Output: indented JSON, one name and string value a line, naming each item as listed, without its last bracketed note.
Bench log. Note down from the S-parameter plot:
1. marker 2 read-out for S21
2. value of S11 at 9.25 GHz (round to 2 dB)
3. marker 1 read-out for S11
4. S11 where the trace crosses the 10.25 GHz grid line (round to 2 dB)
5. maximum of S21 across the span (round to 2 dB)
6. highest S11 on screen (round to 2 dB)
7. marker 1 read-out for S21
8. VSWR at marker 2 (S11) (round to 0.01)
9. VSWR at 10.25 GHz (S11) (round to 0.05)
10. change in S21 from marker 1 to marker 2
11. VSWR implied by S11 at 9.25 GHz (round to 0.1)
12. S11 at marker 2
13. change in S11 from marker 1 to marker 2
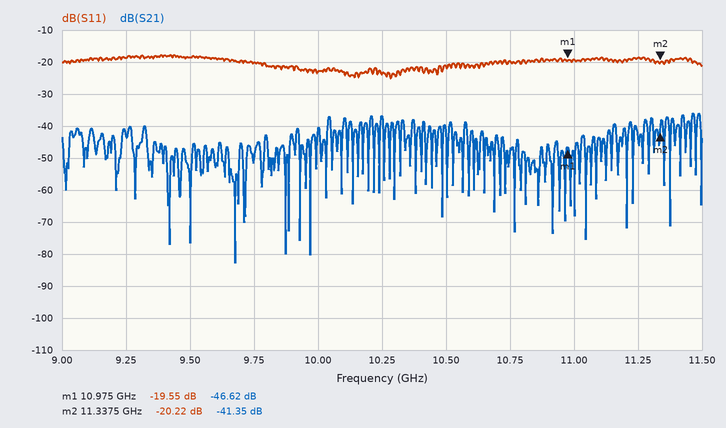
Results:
{
  "marker 2 read-out for S21": "-41.35 dB",
  "value of S11 at 9.25 GHz": "-18 dB",
  "marker 1 read-out for S11": "-19.55 dB",
  "S11 where the trace crosses the 10.25 GHz grid line": "-24 dB",
  "maximum of S21 across the span": "-36 dB",
  "highest S11 on screen": "-18 dB",
  "marker 1 read-out for S21": "-46.62 dB",
  "VSWR at marker 2 (S11)": "1.22",
  "VSWR at 10.25 GHz (S11)": "1.15",
  "change in S21 from marker 1 to marker 2": "5.27 dB",
  "VSWR implied by S11 at 9.25 GHz": "1.3",
  "S11 at marker 2": "-20.22 dB",
  "change in S11 from marker 1 to marker 2": "-0.67 dB"
}
